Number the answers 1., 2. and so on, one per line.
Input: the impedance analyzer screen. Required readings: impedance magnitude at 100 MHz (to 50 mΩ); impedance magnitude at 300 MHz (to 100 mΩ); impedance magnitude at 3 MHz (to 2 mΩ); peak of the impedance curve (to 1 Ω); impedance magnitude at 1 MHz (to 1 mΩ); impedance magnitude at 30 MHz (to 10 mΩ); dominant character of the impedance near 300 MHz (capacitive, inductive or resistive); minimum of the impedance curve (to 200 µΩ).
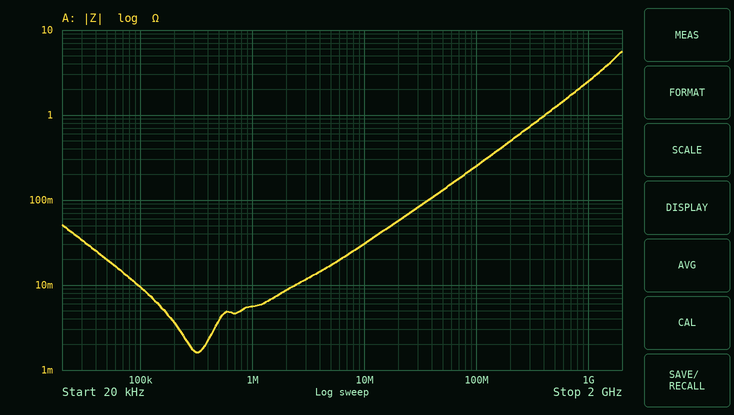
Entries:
1. 250 mΩ
2. 700 mΩ
3. 12 mΩ
4. 6 Ω
5. 6 mΩ
6. 80 mΩ
7. inductive
8. 1.6 mΩ
